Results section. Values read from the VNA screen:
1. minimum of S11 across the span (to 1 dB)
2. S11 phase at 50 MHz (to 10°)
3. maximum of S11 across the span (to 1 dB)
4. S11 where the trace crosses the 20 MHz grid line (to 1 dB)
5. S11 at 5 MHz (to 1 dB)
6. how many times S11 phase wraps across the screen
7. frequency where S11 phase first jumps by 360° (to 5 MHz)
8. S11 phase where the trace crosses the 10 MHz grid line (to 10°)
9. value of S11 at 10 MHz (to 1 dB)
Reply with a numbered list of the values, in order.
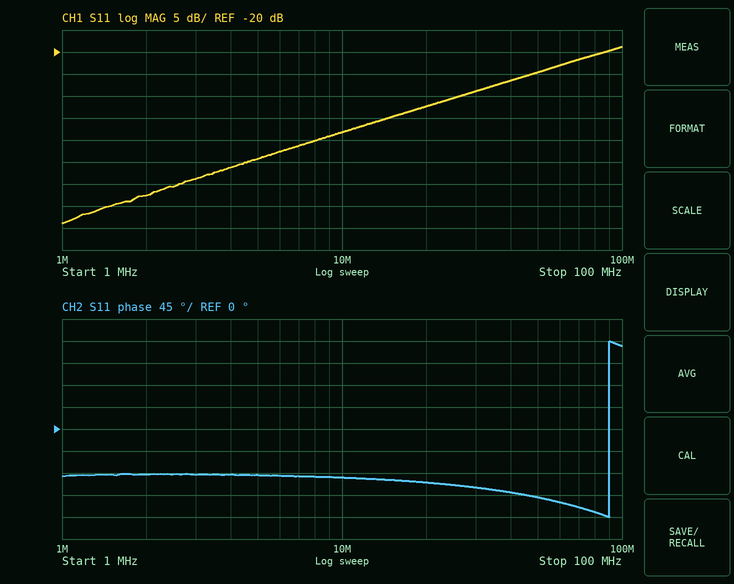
1. -59 dB
2. -140°
3. -19 dB
4. -32 dB
5. -44 dB
6. 1
7. 90 MHz
8. -100°
9. -38 dB
